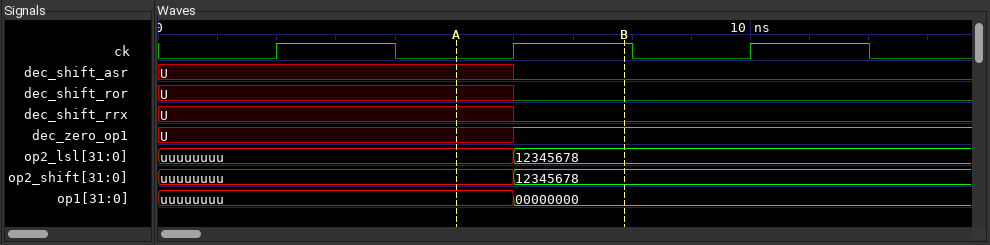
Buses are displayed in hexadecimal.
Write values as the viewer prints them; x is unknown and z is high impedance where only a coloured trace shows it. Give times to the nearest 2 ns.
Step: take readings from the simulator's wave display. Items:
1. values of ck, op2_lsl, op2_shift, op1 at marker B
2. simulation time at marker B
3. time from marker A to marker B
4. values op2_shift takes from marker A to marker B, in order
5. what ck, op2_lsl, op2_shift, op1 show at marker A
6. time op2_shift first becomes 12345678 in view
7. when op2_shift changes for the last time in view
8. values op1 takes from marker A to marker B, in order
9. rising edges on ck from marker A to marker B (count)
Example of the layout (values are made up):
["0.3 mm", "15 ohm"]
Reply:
["ck=1, op2_lsl=12345678, op2_shift=12345678, op1=00000000", "8 ns", "2 ns", "uuuuuuuu, 12345678", "ck=0, op2_lsl=uuuuuuuu, op2_shift=uuuuuuuu, op1=uuuuuuuu", "6 ns", "6 ns", "uuuuuuuu, 00000000", "1"]
